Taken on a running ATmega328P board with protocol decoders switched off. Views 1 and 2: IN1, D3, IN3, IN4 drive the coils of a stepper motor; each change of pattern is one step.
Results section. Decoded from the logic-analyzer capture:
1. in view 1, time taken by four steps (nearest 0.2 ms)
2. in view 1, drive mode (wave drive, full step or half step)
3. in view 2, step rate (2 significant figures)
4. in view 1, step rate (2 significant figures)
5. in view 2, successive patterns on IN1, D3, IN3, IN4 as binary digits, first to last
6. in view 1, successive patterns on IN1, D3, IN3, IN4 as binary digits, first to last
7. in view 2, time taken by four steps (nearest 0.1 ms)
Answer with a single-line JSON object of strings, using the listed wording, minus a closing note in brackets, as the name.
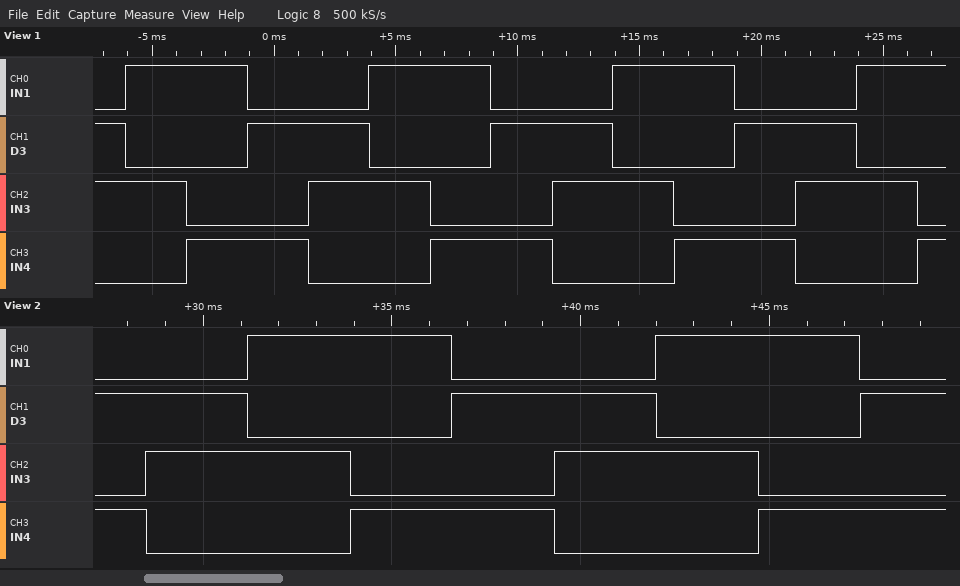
{"in view 1, time taken by four steps": "10.0 ms", "in view 1, drive mode": "full step", "in view 2, step rate": "370 steps/s", "in view 1, step rate": "400 steps/s", "in view 2, successive patterns on IN1, D3, IN3, IN4 as binary digits, first to last": "0101 0110 1010 1001 0101 0110 1010 1001 0101", "in view 1, successive patterns on IN1, D3, IN3, IN4 as binary digits, first to last": "0110 1010 1001 0101 0110 1010 1001 0101 0110 1010 1001 0101 0110 1010 1001", "in view 2, time taken by four steps": "10.8 ms"}
